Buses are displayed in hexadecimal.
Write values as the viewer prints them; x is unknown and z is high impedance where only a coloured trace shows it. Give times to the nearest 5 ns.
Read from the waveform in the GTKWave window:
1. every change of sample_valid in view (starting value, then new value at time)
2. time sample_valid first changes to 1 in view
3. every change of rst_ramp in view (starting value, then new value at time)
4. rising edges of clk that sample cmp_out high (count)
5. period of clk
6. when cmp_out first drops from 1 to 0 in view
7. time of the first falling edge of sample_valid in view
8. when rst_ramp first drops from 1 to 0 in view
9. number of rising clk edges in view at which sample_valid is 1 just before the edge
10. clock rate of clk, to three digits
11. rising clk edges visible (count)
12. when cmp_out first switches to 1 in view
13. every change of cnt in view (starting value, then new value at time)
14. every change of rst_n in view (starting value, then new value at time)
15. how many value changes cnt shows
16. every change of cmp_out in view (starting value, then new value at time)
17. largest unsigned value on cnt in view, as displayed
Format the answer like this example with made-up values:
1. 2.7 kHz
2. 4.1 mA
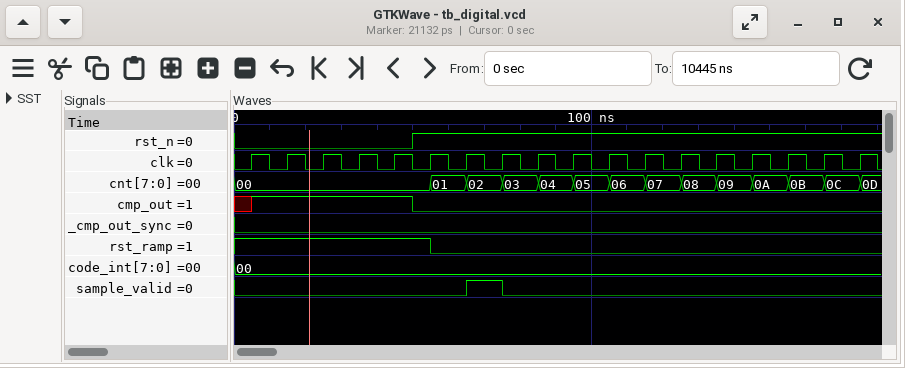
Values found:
1. 0, 1 at 65 ns, 0 at 75 ns
2. 65 ns
3. 1, 0 at 55 ns
4. 4
5. 10 ns
6. 50 ns
7. 75 ns
8. 55 ns
9. 1
10. 100 MHz
11. 18
12. 5 ns
13. 00, 01 at 55 ns, 02 at 65 ns, 03 at 75 ns, 04 at 85 ns, 05 at 95 ns, 06 at 105 ns, 07 at 115 ns, 08 at 125 ns, 09 at 135 ns, 0A at 145 ns, 0B at 155 ns, 0C at 165 ns, 0D at 175 ns
14. 0, 1 at 50 ns
15. 13
16. x, 1 at 5 ns, 0 at 50 ns
17. 0D
